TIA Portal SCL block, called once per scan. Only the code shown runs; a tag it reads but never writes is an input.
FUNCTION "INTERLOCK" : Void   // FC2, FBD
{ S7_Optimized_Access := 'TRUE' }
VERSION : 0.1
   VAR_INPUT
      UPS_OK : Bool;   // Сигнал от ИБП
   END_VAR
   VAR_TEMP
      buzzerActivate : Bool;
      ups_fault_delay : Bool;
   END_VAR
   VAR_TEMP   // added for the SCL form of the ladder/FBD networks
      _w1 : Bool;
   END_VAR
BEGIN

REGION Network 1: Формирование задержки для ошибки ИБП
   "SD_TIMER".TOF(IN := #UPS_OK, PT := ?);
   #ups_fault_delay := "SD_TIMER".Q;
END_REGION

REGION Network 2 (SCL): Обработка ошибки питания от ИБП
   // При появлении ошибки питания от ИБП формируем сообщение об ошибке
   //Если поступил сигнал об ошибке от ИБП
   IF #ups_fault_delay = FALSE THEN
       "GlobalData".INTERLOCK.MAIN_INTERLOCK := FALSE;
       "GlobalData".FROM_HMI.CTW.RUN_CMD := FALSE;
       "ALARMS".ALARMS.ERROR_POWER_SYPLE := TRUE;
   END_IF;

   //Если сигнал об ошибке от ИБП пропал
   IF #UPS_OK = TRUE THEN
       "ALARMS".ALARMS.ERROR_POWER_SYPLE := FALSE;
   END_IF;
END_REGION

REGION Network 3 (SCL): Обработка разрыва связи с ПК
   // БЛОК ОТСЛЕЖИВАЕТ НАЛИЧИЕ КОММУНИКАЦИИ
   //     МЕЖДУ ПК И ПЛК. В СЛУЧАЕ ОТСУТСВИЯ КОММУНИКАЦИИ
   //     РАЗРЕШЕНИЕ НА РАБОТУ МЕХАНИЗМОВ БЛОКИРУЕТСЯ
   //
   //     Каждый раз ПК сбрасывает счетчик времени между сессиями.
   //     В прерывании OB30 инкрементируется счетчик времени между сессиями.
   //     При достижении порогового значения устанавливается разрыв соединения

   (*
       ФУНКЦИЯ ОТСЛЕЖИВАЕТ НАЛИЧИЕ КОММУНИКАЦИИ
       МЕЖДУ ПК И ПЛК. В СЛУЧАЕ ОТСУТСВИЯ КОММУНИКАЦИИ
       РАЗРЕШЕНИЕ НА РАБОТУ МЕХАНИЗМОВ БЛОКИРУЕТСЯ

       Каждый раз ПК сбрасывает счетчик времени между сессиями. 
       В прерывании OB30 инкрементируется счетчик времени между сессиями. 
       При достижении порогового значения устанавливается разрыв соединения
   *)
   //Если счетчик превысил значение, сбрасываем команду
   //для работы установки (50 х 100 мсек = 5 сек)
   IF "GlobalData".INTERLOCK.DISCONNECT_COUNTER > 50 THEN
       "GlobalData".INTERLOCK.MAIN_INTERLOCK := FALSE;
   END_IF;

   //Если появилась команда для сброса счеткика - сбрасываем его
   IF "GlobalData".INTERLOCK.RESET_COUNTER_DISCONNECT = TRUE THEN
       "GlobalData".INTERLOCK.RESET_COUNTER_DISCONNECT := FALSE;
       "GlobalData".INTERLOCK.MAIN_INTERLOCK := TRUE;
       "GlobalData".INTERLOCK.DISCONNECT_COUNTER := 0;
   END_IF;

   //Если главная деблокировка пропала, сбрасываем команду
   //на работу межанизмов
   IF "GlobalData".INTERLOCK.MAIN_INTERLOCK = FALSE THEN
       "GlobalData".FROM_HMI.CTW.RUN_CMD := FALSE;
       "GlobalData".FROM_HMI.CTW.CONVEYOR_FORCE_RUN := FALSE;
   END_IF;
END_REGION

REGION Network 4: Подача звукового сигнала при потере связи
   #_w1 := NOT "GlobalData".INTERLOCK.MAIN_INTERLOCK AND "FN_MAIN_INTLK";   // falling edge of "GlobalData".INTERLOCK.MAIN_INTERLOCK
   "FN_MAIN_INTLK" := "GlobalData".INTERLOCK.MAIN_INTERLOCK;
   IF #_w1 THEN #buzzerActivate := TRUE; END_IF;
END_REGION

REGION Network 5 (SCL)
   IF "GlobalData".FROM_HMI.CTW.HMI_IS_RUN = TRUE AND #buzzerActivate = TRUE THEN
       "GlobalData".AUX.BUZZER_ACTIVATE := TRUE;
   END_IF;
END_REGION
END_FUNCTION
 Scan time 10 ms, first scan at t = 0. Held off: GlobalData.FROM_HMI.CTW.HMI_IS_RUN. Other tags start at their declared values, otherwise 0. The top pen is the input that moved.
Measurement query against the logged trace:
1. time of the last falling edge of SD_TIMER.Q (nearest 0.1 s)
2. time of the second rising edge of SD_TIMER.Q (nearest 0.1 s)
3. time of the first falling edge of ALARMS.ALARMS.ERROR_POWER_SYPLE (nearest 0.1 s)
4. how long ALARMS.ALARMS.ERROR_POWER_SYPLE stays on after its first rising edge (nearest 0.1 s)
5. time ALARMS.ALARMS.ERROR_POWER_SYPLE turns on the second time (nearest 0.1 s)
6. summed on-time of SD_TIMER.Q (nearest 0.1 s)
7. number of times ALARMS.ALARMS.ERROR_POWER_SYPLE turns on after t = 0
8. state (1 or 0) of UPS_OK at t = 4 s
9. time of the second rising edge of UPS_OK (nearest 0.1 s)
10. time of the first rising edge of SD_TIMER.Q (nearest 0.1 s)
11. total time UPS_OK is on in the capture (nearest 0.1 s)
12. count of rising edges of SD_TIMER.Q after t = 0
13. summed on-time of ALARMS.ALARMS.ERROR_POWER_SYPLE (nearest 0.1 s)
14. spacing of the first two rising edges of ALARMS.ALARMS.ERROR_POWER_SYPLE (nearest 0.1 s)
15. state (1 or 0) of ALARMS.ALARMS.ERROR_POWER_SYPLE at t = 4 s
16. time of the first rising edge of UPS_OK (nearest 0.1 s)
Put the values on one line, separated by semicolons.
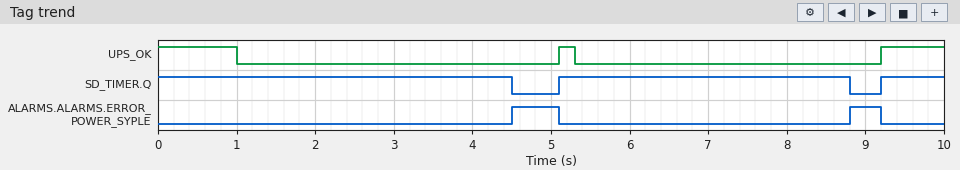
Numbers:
8.8 s; 9.2 s; 5.1 s; 0.6 s; 8.8 s; 9.0 s; 2; 0; 9.2 s; 5.1 s; 2.0 s; 2; 1.0 s; 4.3 s; 0; 5.1 s
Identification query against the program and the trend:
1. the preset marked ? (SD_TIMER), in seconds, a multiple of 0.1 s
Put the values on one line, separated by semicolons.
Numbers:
3.5 s
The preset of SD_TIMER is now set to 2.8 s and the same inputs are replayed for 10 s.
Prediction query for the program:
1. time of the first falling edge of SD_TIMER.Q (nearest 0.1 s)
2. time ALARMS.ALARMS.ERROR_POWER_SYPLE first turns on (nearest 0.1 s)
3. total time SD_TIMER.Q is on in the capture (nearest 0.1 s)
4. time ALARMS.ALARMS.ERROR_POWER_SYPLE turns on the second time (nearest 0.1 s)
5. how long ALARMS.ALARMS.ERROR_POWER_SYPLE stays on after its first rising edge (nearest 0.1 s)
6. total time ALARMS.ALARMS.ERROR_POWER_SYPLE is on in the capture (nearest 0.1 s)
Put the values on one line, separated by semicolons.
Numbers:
3.8 s; 3.8 s; 7.6 s; 8.1 s; 1.3 s; 2.4 s
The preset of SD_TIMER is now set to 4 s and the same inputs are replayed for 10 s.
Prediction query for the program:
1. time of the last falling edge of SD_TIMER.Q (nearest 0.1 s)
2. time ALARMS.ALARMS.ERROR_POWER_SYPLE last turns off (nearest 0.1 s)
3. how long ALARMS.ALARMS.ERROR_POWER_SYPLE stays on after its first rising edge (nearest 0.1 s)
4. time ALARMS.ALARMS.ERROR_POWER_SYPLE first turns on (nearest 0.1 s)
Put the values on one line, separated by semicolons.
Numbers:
5.0 s; 5.1 s; 0.1 s; 5.0 s
